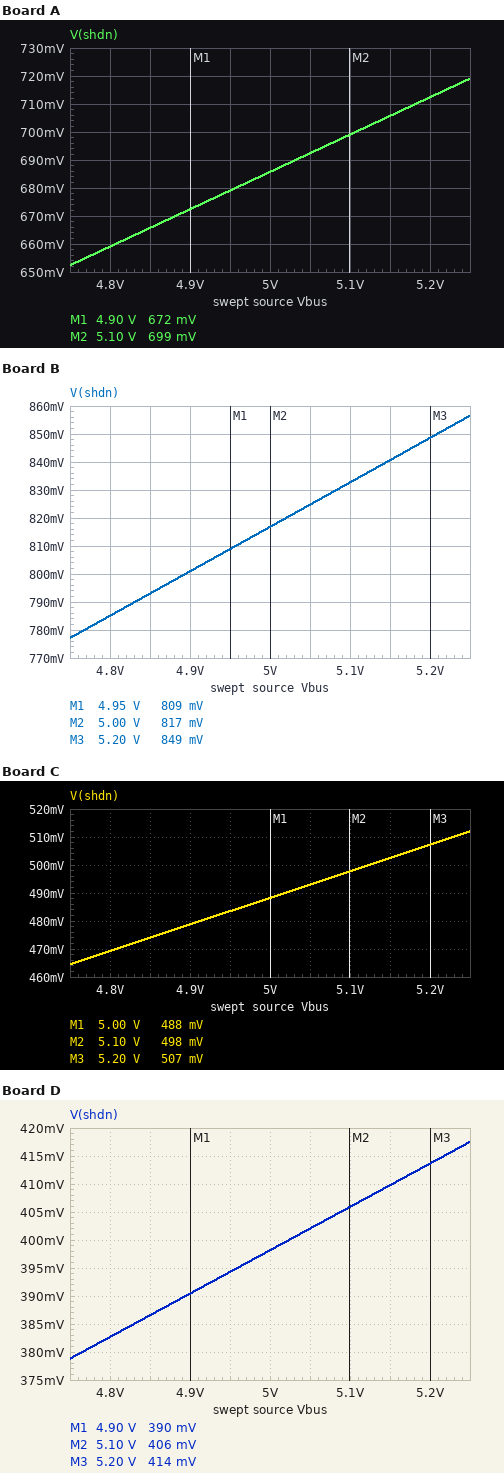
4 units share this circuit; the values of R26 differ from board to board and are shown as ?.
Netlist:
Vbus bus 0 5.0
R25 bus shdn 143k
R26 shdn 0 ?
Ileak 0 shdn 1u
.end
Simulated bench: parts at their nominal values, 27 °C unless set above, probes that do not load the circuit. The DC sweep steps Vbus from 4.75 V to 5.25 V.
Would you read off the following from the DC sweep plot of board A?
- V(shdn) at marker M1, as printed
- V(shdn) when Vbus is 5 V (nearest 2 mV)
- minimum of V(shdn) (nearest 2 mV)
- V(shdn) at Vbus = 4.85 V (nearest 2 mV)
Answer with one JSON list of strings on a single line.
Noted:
["672 mV", "686 mV", "652 mV", "666 mV"]
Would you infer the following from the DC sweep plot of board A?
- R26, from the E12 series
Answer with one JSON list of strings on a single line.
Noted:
["22 kΩ"]
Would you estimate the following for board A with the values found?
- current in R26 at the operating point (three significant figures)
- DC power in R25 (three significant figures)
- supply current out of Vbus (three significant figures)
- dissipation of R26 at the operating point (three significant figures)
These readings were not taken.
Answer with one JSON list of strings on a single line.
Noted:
["31.2 µA", "130 µW", "30.2 µA", "21.4 µW"]
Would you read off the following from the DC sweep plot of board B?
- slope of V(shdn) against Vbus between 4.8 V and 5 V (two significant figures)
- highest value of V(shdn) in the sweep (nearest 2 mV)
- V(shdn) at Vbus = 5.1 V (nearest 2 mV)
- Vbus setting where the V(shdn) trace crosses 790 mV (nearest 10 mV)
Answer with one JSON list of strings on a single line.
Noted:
["0.16 V/V", "856 mV", "832 mV", "4.83 V"]
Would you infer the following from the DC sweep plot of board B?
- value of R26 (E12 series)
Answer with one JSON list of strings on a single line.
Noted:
["27 kΩ"]
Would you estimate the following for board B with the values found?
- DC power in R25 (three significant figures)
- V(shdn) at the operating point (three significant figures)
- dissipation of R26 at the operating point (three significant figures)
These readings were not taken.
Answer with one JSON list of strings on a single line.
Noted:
["122 µW", "817 mV", "24.7 µW"]
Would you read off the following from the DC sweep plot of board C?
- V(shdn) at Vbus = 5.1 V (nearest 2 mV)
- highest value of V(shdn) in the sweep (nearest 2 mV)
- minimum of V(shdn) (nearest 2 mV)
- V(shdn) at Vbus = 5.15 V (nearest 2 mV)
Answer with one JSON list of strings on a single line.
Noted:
["498 mV", "512 mV", "464 mV", "502 mV"]
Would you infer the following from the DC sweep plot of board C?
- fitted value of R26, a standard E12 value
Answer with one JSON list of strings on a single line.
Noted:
["15 kΩ"]
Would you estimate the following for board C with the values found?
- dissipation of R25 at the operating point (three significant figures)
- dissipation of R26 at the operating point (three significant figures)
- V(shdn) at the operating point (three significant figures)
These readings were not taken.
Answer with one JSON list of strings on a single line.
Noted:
["142 µW", "15.9 µW", "488 mV"]
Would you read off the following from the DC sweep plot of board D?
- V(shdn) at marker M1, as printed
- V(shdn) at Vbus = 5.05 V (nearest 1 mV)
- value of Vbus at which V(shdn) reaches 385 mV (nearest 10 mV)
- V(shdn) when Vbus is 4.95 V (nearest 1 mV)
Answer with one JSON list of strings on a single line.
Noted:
["390 mV", "402 mV", "4.83 V", "394 mV"]
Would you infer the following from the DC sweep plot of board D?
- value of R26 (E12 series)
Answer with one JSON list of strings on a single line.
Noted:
["12 kΩ"]
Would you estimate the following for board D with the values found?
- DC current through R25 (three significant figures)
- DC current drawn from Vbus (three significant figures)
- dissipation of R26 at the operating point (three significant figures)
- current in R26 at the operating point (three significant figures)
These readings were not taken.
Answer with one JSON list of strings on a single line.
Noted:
["32.2 µA", "32.2 µA", "13.2 µW", "33.2 µA"]
